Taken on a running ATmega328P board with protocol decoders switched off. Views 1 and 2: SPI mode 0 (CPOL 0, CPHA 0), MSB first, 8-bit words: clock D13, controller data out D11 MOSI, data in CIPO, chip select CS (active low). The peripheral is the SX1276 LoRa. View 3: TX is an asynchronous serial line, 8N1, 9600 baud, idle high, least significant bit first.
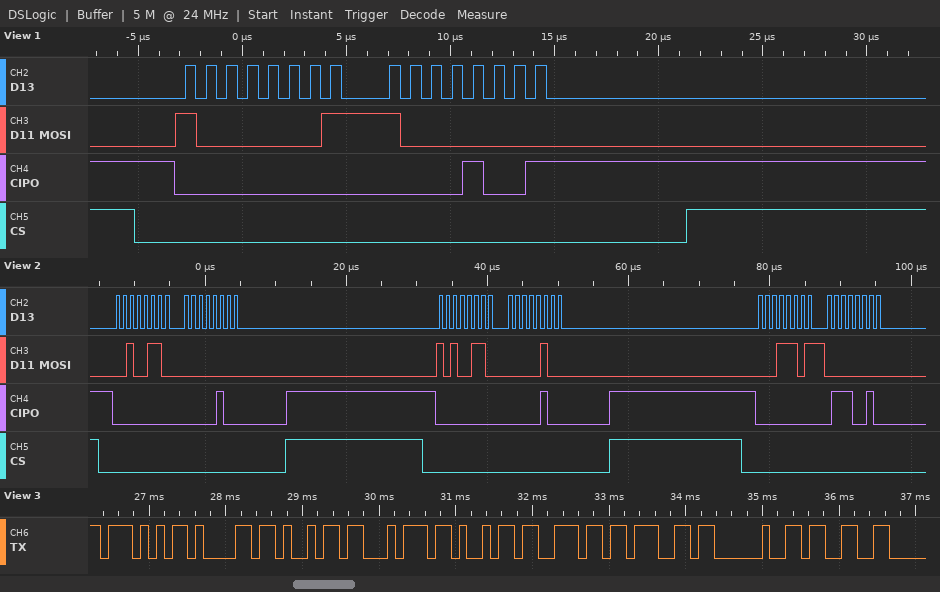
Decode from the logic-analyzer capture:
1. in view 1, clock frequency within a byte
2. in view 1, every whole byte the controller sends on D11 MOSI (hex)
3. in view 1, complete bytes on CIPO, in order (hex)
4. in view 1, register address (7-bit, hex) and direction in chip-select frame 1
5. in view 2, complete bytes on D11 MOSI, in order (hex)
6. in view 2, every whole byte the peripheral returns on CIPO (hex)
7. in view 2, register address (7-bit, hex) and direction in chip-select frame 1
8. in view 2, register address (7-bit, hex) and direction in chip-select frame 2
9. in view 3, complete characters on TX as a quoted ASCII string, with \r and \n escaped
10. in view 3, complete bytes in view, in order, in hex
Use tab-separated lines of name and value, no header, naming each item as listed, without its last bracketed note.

in view 1, clock frequency within a byte	1 MHz
in view 1, every whole byte the controller sends on D11 MOSI	81 80
in view 1, complete bytes on CIPO, in order	00 09
in view 1, register address (7-bit, hex) and direction in chip-select frame 1	0x01 write
in view 2, complete bytes on D11 MOSI, in order	0x26 0x00 0xA6 0x04 0x1D 0x00
in view 2, every whole byte the peripheral returns on CIPO	0x00 0x04 0x00 0x04 0x00 0x72
in view 2, register address (7-bit, hex) and direction in chip-select frame 1	0x26 read
in view 2, register address (7-bit, hex) and direction in chip-select frame 2	0x26 write
in view 3, complete characters on TX as a quoted ASCII string, with \r and \n escaped	"Waiting 3"
in view 3, complete bytes in view, in order, in hex	0x57 0x61 0x69 0x74 0x69 0x6E 0x67 0x20 0x33
